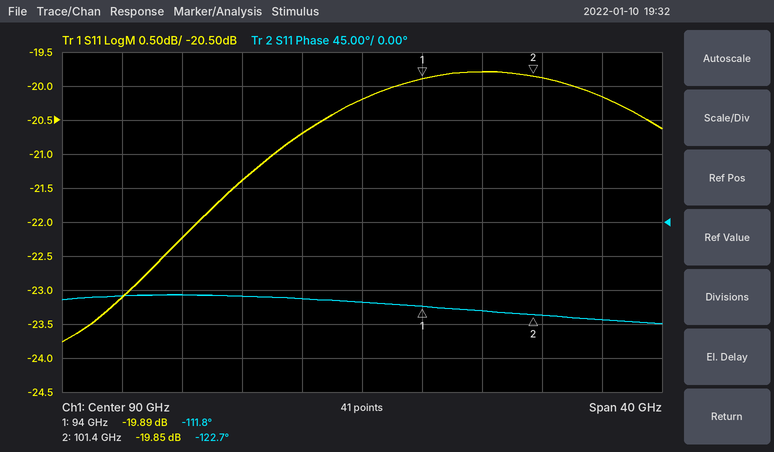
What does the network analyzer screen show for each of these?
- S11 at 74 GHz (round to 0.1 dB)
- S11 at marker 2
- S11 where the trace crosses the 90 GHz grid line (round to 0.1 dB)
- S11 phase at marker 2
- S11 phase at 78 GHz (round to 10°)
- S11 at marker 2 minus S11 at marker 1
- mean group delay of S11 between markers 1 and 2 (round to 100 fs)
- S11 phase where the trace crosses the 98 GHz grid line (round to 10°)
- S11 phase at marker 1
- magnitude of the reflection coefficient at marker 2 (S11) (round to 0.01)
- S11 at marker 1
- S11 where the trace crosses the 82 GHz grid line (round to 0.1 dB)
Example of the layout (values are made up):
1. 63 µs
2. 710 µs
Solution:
1. -23.1 dB
2. -19.85 dB
3. -20.2 dB
4. -122.7°
5. -100°
6. 0.04 dB
7. 4.1 ps
8. -120°
9. -111.8°
10. 0.10
11. -19.89 dB
12. -21.4 dB
